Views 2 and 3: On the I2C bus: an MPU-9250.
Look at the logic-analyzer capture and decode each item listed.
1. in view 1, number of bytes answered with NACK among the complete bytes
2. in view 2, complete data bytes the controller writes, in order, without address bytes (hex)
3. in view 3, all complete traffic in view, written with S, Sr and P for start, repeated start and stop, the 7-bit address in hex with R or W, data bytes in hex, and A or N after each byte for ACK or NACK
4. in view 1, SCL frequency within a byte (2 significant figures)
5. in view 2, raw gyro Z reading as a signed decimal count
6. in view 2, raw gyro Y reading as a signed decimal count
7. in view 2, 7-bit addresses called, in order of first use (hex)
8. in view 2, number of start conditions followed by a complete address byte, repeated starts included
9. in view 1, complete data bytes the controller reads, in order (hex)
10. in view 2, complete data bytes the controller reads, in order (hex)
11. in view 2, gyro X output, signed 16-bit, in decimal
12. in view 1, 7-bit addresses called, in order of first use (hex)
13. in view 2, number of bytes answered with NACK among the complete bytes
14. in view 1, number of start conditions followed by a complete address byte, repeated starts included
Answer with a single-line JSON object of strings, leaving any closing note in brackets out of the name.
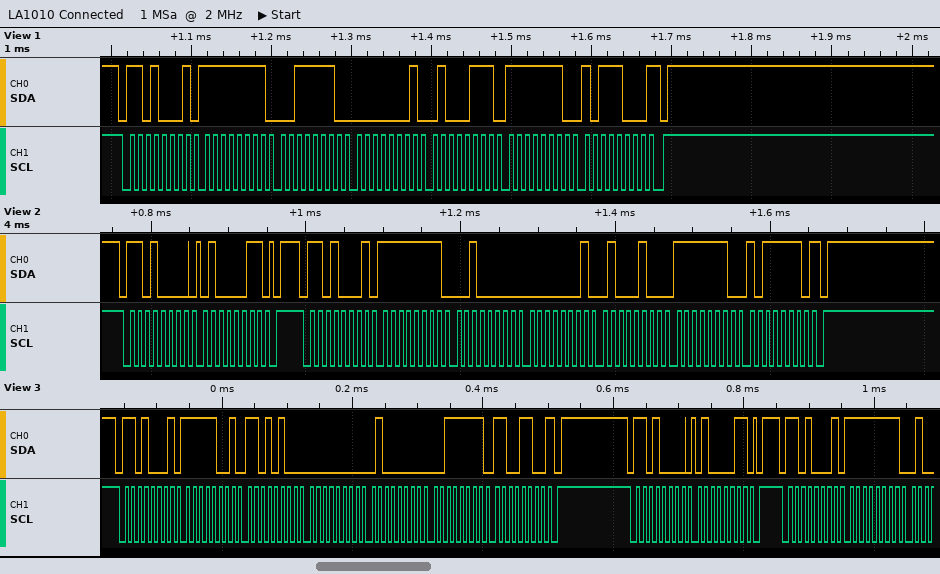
{"in view 1, number of bytes answered with NACK among the complete bytes": "1", "in view 2, complete data bytes the controller writes, in order, without address bytes": "43", "in view 3, all complete traffic in view, written with S, Sr and P for start, repeated start and stop, the 7-bit address in hex with R or W, data bytes in hex, and A or N after each byte for ACK or NACK": "S 68R A F9 A D4 A 00 A 40 A 3F A CC N P S 68W A 43 A P S 68R A FF A", "in view 1, SCL frequency within a byte": "100 kHz", "in view 2, raw gyro Z reading as a signed decimal count": "-322", "in view 2, raw gyro Y reading as a signed decimal count": "324", "in view 2, 7-bit addresses called, in order of first use": "0x68", "in view 2, number of start conditions followed by a complete address byte, repeated starts included": "2", "in view 1, complete data bytes the controller reads, in order": "FF 3E 01 47 FE B8", "in view 2, complete data bytes the controller reads, in order": "FF 20 01 44 FE BE", "in view 2, gyro X output, signed 16-bit, in decimal": "-224", "in view 1, 7-bit addresses called, in order of first use": "0x68", "in view 2, number of bytes answered with NACK among the complete bytes": "1", "in view 1, number of start conditions followed by a complete address byte, repeated starts included": "1"}
